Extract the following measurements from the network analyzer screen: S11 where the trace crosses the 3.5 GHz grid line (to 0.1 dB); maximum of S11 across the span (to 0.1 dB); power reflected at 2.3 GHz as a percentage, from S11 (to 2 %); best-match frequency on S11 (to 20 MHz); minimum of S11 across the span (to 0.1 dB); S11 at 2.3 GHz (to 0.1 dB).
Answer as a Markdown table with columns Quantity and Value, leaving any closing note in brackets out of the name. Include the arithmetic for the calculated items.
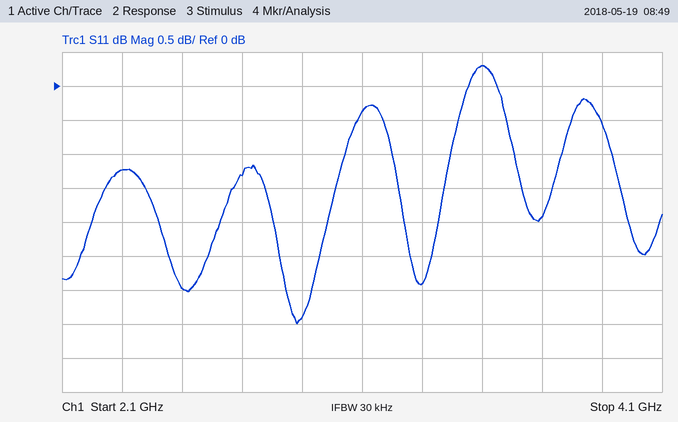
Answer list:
| Quantity | Value |
|---|---|
| S11 where the trace crosses the 3.5 GHz grid line | 0.3 dB |
| maximum of S11 across the span | 0.3 dB |
| power reflected at 2.3 GHz as a percentage, from S11 | 10^(-1.2/10) ≈ 76 % |
| best-match frequency on S11 | 2.88 GHz |
| minimum of S11 across the span | -3.5 dB |
| S11 at 2.3 GHz | -1.2 dB |
